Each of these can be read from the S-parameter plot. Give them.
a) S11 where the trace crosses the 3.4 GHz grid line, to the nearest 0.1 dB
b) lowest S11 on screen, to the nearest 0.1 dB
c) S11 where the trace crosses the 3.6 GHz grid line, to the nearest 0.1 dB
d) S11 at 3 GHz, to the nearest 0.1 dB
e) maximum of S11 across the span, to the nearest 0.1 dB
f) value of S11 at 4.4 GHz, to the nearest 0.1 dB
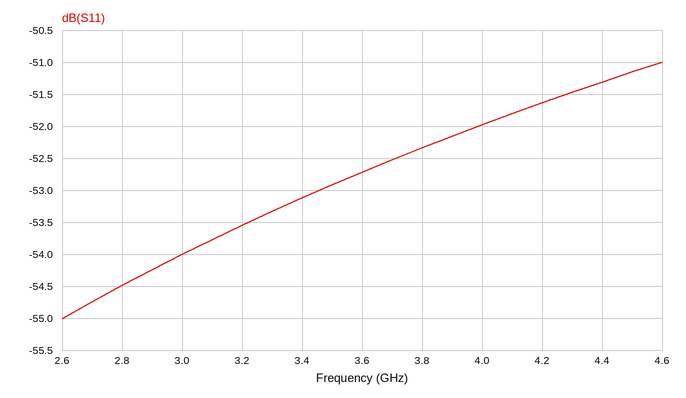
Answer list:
-53.1 dB
-55.0 dB
-52.7 dB
-54.0 dB
-51.0 dB
-51.3 dB
